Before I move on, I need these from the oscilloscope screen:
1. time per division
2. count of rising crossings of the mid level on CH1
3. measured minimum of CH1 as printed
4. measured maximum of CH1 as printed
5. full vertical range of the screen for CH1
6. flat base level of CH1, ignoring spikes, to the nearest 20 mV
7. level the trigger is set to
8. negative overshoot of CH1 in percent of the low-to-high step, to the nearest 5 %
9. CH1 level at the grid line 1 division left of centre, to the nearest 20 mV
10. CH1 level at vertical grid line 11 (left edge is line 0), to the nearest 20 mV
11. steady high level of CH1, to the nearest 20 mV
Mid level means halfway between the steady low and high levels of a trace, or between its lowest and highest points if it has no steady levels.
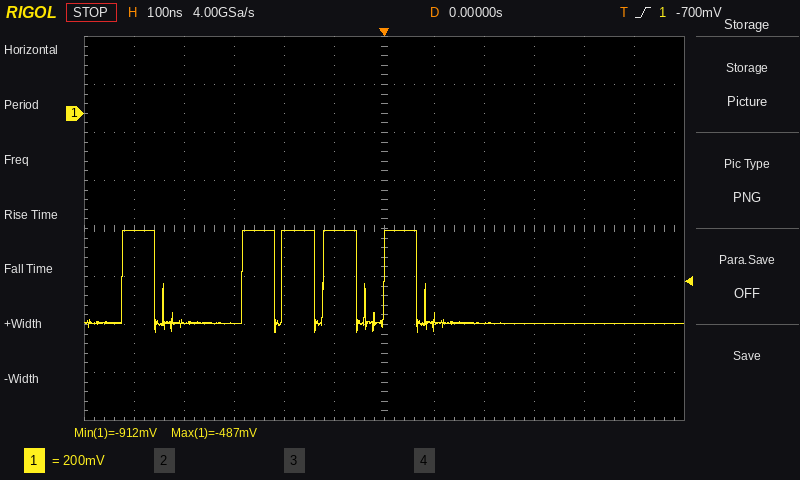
100 ns
5
-912 mV
-487 mV
1.6 V
-880 mV
-700 mV
10 %
-480 mV
-880 mV
-480 mV
